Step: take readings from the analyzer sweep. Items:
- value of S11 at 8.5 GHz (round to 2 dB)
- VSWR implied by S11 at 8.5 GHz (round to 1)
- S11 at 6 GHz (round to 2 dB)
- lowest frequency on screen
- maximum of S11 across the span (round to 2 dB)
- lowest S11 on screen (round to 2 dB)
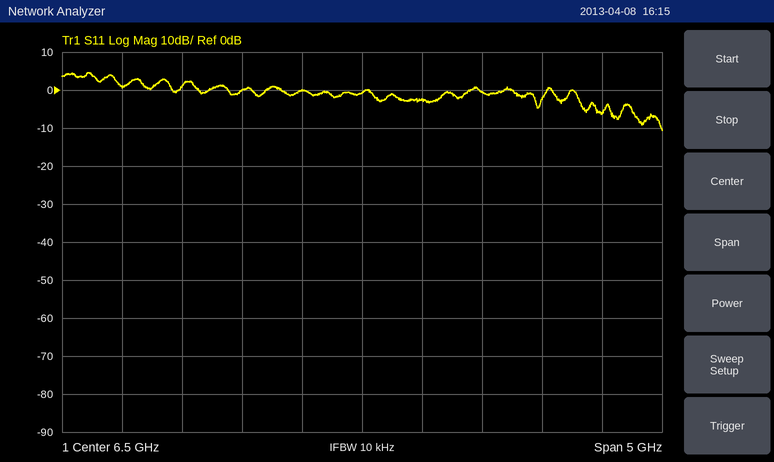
-6 dB
3
0 dB
4 GHz
4 dB
-10 dB
